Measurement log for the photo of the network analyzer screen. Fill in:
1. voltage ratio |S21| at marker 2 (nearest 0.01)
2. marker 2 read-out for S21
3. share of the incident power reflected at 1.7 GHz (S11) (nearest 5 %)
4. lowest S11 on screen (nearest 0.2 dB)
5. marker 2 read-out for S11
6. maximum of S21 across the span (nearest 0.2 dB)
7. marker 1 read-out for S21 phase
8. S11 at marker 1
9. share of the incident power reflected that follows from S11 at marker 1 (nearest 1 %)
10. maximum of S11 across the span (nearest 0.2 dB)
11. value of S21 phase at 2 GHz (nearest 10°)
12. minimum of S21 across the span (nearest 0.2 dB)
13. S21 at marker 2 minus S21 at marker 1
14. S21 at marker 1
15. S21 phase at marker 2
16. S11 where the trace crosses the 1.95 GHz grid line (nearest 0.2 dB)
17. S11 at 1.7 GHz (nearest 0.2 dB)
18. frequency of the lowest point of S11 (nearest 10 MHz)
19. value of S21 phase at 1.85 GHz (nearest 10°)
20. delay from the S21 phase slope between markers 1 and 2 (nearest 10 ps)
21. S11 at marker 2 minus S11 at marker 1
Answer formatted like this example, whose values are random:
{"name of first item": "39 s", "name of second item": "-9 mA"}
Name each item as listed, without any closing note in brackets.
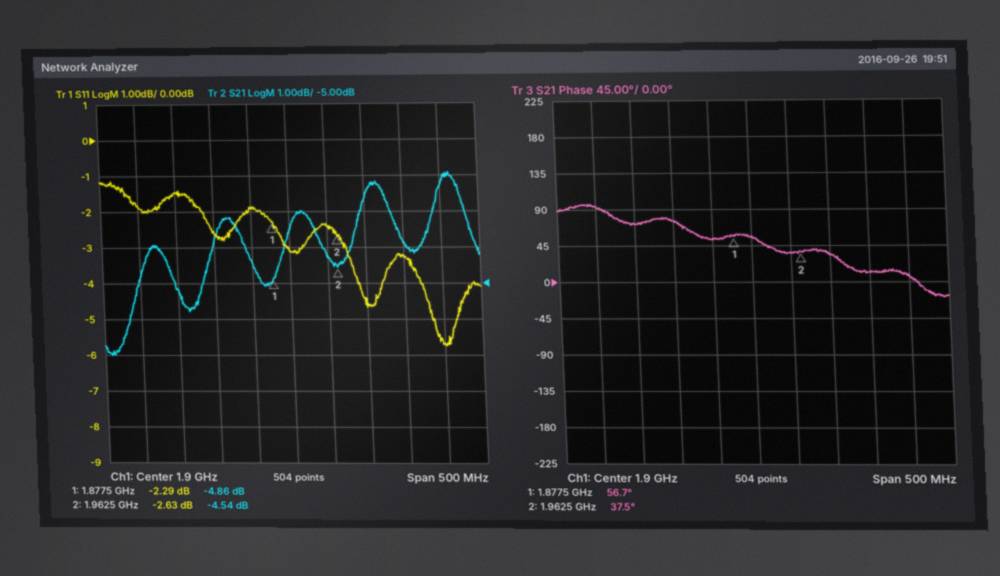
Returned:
{"voltage ratio |S21| at marker 2": "0.59", "marker 2 read-out for S21": "-4.54 dB", "share of the incident power reflected at 1.7 GHz (S11)": "65 %", "lowest S11 on screen": "-5.8 dB", "marker 2 read-out for S11": "-2.63 dB", "maximum of S21 across the span": "-2.0 dB", "marker 1 read-out for S21 phase": "56.7°", "S11 at marker 1": "-2.29 dB", "share of the incident power reflected that follows from S11 at marker 1": "59 %", "maximum of S11 across the span": "-1.2 dB", "value of S21 phase at 2 GHz": "30°", "minimum of S21 across the span": "-7.0 dB", "S21 at marker 2 minus S21 at marker 1": "0.32 dB", "S21 at marker 1": "-4.86 dB", "S21 phase at marker 2": "37.5°", "S11 where the trace crosses the 1.95 GHz grid line": "-2.4 dB", "S11 at 1.7 GHz": "-1.8 dB", "frequency of the lowest point of S11": "2.10 GHz", "value of S21 phase at 1.85 GHz": "50°", "delay from the S21 phase slope between markers 1 and 2": "630 ps", "S11 at marker 2 minus S11 at marker 1": "-0.34 dB"}
